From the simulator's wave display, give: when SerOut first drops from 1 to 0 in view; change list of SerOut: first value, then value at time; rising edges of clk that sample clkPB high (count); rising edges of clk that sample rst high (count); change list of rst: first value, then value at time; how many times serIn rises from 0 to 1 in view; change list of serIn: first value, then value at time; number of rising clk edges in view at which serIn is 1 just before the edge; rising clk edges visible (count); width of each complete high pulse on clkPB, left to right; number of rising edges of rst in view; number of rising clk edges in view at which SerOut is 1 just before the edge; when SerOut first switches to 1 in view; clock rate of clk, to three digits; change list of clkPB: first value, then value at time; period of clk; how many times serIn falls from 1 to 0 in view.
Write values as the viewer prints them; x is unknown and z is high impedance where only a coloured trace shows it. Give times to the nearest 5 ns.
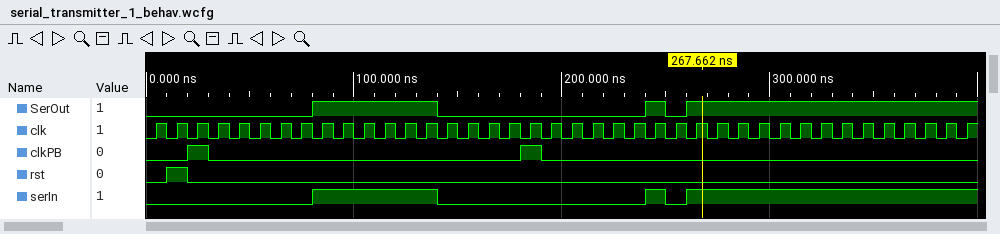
140 ns
0, 1 at 80 ns, 0 at 140 ns, 1 at 240 ns, 0 at 250 ns, 1 at 260 ns
2
1
0, 1 at 10 ns, 0 at 20 ns
3
0, 1 at 80 ns, 0 at 140 ns, 1 at 240 ns, 0 at 250 ns, 1 at 260 ns
21
40
10 ns, 10 ns
1
21
80 ns
100 MHz
0, 1 at 20 ns, 0 at 30 ns, 1 at 180 ns, 0 at 190 ns
10 ns
2
